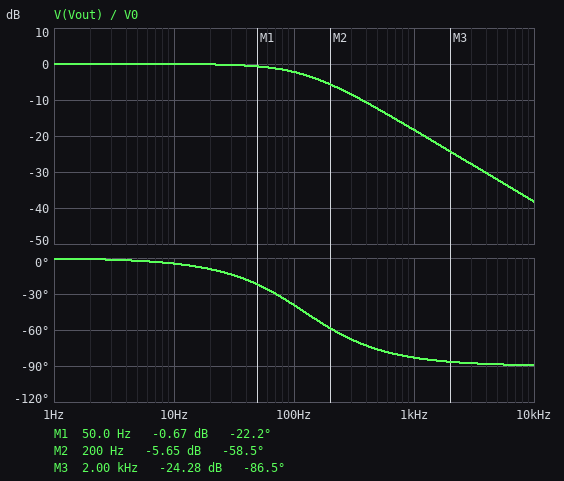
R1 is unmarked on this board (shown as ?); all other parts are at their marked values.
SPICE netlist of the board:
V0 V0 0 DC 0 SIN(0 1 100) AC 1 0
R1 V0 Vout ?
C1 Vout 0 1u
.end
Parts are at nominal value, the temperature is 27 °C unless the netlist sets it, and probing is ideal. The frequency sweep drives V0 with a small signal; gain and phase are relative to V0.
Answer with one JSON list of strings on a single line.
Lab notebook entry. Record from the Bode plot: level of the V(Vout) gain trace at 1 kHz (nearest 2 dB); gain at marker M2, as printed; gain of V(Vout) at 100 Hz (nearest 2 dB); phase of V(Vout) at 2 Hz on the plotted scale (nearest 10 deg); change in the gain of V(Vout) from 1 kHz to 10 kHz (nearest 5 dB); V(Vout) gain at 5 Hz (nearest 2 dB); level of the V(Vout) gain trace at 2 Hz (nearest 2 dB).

["-18 dB", "-5.65 dB", "-2 dB", "0 deg", "-20 dB", "0 dB", "0 dB"]
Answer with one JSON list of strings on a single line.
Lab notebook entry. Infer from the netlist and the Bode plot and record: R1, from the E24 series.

["1.3 kΩ"]
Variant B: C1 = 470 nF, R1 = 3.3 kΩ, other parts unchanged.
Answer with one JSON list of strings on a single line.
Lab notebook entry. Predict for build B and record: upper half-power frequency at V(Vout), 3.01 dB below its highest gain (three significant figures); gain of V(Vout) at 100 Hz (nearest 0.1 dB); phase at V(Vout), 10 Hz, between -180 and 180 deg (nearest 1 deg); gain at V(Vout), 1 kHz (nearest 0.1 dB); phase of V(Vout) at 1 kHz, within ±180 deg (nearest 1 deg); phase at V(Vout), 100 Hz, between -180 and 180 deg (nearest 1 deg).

["103 Hz", "-2.9 dB", "-6 deg", "-19.8 dB", "-84 deg", "-44 deg"]
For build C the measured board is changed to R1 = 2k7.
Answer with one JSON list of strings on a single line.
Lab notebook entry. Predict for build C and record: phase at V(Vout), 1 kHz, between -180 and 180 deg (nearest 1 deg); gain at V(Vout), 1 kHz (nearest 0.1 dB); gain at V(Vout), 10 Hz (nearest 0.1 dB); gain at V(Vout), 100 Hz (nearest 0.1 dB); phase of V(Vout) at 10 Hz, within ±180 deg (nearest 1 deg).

["-87 deg", "-24.6 dB", "-0.1 dB", "-5.9 dB", "-10 deg"]
